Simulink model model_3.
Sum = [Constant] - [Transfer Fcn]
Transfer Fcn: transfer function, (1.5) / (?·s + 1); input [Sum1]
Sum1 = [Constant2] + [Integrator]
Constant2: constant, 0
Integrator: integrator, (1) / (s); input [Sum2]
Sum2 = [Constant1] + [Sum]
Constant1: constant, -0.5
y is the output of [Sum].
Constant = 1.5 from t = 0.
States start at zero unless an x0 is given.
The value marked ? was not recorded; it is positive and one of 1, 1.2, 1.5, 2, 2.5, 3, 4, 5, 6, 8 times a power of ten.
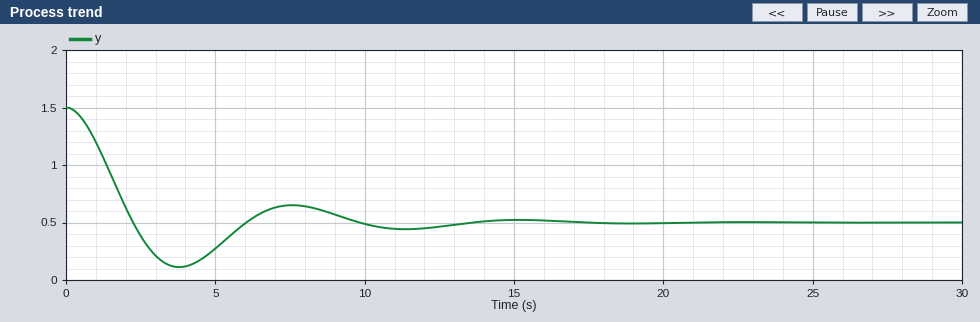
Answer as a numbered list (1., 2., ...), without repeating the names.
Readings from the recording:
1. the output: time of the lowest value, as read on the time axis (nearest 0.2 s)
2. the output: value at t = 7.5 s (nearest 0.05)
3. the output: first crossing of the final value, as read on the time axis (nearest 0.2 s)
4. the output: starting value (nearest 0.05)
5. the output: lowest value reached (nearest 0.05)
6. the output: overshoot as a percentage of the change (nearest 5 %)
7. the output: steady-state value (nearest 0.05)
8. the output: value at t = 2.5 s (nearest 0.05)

1. 3.8 s
2. 0.65
3. 2.2 s
4. 1.50
5. 0.10
6. 40 %
7. 0.50
8. 0.40
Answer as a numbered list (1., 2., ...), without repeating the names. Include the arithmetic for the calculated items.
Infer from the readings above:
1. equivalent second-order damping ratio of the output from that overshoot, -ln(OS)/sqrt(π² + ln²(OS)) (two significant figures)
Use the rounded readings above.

1. ln(0.4) = -0.916; 0.916 / sqrt(9.870 + 0.840) = 0.28
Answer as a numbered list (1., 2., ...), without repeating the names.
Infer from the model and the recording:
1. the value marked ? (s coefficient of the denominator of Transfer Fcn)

1. 2
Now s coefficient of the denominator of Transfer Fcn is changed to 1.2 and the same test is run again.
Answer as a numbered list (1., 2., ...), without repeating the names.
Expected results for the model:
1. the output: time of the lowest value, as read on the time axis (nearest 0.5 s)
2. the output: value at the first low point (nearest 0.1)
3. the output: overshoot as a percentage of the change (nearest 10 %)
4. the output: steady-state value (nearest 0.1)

1. 3.0 s
2. 0.2
3. 30 %
4. 0.5
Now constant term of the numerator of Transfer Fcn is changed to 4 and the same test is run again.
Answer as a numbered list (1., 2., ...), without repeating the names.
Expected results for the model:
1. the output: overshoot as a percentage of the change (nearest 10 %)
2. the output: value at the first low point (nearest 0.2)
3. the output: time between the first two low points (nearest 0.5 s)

1. 60 %
2. 0.0
3. 4.5 s
